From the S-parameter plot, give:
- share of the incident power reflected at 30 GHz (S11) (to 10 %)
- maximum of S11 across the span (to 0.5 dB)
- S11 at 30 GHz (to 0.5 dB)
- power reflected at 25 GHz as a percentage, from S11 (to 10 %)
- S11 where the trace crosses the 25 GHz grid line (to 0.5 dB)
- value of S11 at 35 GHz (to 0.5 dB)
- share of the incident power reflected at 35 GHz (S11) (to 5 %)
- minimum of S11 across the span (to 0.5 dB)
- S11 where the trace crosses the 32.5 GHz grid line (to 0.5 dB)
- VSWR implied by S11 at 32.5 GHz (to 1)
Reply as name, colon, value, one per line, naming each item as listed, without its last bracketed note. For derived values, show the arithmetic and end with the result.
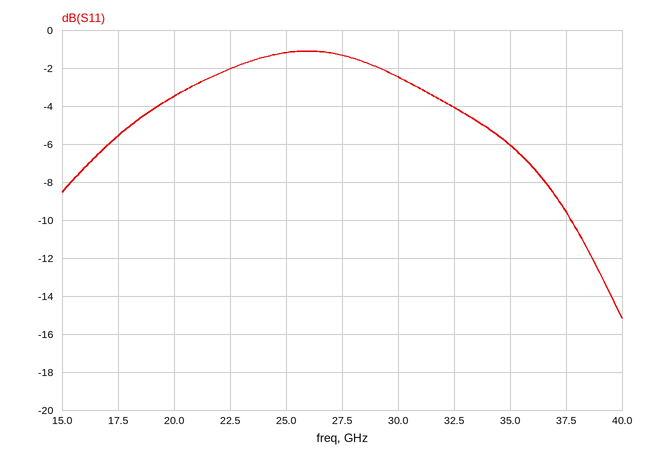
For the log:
share of the incident power reflected at 30 GHz (S11): 10^(-2.5/10) ≈ 56.2 %, so 60 % to the nearest 10 %
maximum of S11 across the span: -1.0 dB
S11 at 30 GHz: -2.5 dB
power reflected at 25 GHz as a percentage, from S11: 10^(-1/10) ≈ 79.4 %, so 80 % to the nearest 10 %
S11 where the trace crosses the 25 GHz grid line: -1.0 dB
value of S11 at 35 GHz: -6.0 dB
share of the incident power reflected at 35 GHz (S11): 10^(-6/10) ≈ 25 %
minimum of S11 across the span: -15.0 dB
S11 where the trace crosses the 32.5 GHz grid line: -4.0 dB
VSWR implied by S11 at 32.5 GHz: |Γ| = 10^(-4/20) = 0.6310; VSWR = (1 + 0.6310)/(1 − 0.6310) ≈ 4
